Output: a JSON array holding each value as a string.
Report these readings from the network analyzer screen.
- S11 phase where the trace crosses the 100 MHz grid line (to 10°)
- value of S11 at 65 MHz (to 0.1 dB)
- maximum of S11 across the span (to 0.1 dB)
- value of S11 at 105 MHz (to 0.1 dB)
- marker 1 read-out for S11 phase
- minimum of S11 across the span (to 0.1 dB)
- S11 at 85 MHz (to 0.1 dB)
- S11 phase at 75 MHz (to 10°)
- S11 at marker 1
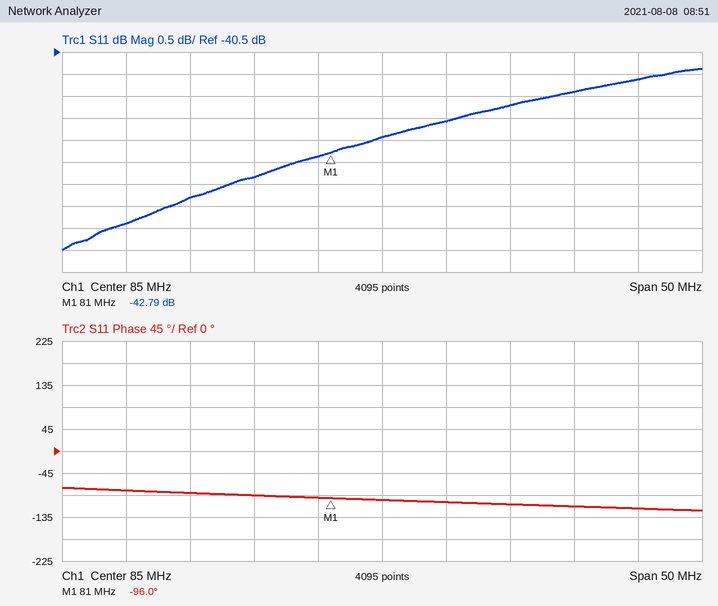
["-110°", "-44.4 dB", "-40.9 dB", "-41.1 dB", "-96.0°", "-45.0 dB", "-42.4 dB", "-90°", "-42.79 dB"]
